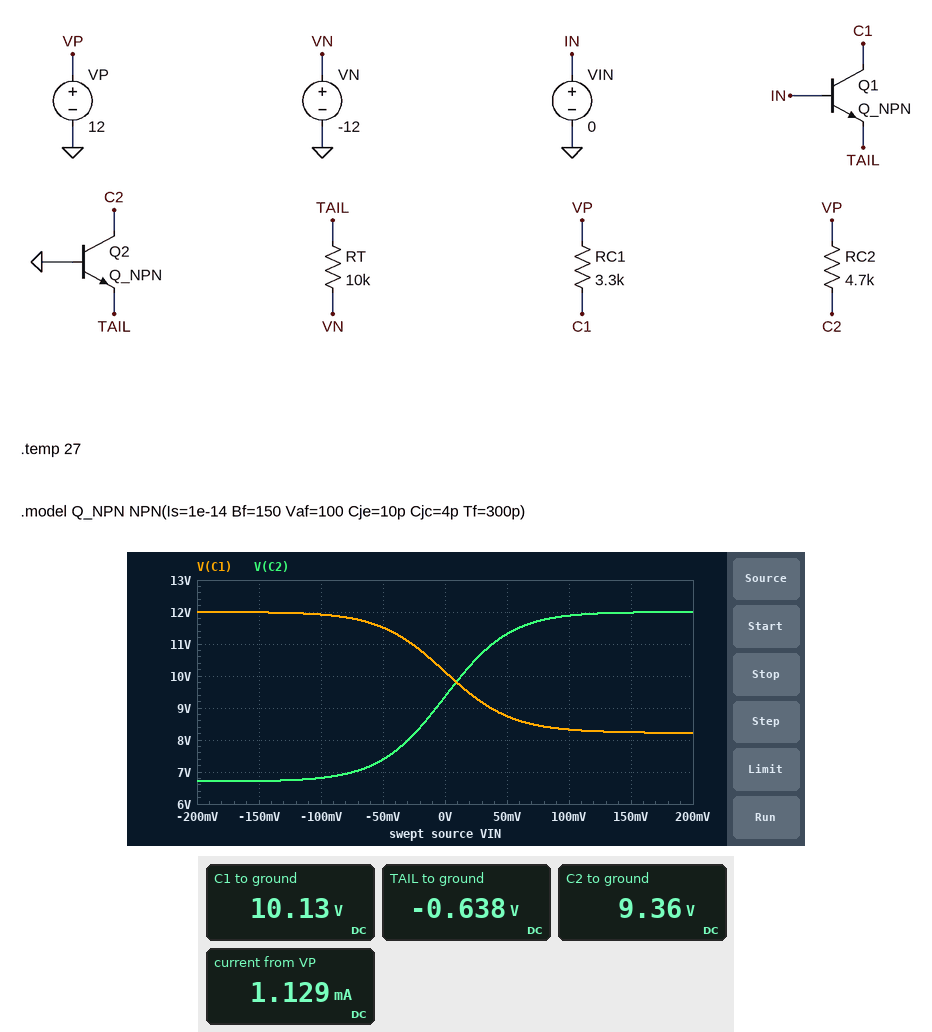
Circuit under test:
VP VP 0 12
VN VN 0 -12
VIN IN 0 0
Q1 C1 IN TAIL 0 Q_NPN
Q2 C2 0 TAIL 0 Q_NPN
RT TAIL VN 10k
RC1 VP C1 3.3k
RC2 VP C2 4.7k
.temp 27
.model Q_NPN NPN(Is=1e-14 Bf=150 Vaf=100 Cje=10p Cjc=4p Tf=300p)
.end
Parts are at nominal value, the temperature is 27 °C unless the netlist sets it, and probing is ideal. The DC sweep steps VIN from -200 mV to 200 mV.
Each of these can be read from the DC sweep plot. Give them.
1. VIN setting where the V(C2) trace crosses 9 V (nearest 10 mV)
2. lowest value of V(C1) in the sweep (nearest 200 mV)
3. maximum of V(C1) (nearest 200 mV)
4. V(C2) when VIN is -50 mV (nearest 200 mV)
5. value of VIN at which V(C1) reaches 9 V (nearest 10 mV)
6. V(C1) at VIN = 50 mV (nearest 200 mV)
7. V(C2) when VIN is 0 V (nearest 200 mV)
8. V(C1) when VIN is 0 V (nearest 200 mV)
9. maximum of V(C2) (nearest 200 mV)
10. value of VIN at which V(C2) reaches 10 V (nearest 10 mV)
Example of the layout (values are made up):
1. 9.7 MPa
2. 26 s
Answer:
1. -10 mV
2. 8.2 V
3. 12.0 V
4. 7.4 V
5. 40 mV
6. 8.8 V
7. 9.4 V
8. 10.2 V
9. 12.0 V
10. 10 mV
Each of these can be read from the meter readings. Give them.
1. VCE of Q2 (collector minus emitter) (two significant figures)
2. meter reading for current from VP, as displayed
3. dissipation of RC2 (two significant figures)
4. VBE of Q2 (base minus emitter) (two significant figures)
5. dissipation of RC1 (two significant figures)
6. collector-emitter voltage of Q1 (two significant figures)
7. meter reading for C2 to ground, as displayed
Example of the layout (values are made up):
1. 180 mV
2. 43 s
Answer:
1. 10 V
2. 1.129 mA
3. 1.5 mW
4. 640 mV
5. 1.1 mW
6. 11 V
7. 9.36 V
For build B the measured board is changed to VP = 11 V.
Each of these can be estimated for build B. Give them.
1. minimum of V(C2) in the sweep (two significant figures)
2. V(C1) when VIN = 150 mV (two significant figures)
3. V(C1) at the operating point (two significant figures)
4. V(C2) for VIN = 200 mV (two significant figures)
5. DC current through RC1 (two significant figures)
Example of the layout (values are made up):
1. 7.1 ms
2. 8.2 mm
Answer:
1. 5.7 V
2. 7.2 V
3. 9.1 V
4. 11 V
5. 570 µA
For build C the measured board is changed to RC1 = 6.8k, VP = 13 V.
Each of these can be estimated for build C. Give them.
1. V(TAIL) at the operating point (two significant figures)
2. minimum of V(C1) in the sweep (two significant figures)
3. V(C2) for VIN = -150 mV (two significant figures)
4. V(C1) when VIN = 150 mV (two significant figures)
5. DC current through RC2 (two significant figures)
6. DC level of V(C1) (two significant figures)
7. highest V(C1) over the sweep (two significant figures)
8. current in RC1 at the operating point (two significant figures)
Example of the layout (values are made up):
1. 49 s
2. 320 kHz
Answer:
1. -640 mV
2. 5.2 V
3. 7.7 V
4. 5.3 V
5. 570 µA
6. 9.2 V
7. 13 V
8. 560 µA
